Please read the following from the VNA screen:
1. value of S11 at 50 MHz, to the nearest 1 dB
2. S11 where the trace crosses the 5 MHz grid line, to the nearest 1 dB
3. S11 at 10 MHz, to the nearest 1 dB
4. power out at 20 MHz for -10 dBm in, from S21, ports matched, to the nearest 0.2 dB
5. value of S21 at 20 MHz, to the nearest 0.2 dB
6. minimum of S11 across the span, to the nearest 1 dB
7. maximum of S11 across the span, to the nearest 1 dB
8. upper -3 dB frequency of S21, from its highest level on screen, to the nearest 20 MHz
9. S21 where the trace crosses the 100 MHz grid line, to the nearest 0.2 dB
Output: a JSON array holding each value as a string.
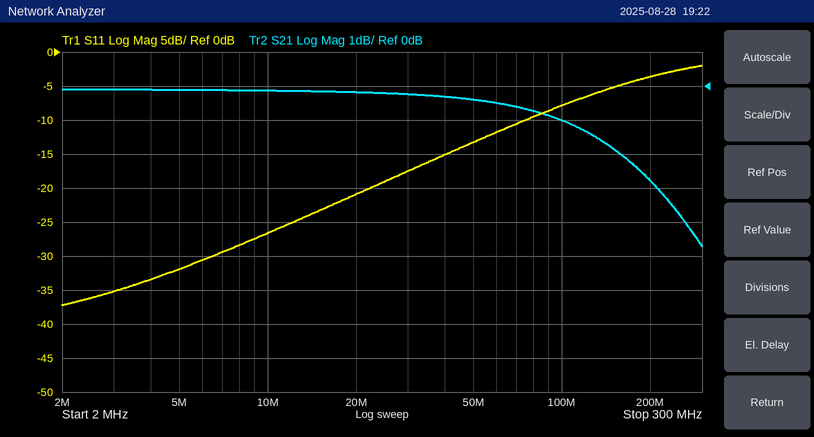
["-13 dB", "-32 dB", "-27 dB", "-10.2 dBm", "-0.2 dB", "-37 dB", "-2 dB", "220 MHz", "-1.0 dB"]
